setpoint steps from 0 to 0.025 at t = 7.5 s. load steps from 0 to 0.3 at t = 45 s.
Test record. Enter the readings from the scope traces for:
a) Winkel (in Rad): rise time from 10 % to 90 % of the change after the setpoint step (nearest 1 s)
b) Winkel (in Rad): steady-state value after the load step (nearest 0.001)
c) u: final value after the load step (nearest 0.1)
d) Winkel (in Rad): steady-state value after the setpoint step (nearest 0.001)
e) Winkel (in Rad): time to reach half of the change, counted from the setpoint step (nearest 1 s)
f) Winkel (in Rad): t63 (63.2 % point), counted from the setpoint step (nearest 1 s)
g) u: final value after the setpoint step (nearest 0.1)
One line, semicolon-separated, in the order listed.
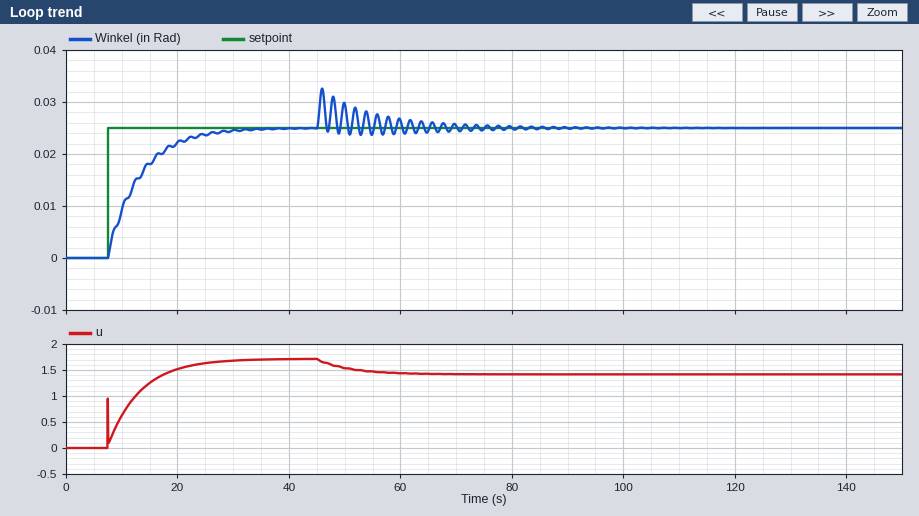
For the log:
12 s; 0.025; 1.4; 0.025; 4 s; 6 s; 1.7
